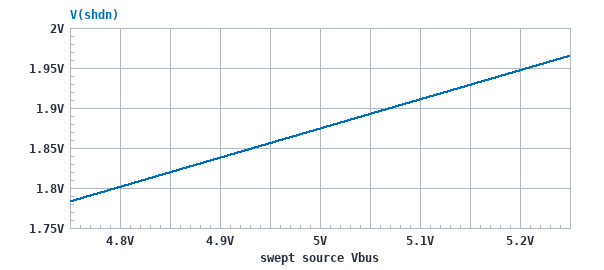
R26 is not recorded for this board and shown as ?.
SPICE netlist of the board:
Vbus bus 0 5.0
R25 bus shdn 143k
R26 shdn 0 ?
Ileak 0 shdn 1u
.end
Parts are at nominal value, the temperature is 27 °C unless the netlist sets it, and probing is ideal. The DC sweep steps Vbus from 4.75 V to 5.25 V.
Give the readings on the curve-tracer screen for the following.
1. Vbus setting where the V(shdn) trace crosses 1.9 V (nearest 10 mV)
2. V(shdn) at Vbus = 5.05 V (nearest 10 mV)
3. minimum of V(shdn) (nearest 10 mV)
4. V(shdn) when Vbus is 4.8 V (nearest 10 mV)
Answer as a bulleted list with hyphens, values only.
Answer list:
- 5.07 V
- 1.89 V
- 1.78 V
- 1.80 V
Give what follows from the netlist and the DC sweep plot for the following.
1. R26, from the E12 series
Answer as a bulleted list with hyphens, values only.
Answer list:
- 82 kΩ
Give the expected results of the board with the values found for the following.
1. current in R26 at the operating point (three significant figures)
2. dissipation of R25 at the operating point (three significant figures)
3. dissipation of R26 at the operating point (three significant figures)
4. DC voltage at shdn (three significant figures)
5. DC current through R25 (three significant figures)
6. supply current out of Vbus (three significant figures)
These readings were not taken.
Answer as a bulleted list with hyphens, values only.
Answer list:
- 22.9 µA
- 68.3 µW
- 42.8 µW
- 1.87 V
- 21.9 µA
- 21.9 µA
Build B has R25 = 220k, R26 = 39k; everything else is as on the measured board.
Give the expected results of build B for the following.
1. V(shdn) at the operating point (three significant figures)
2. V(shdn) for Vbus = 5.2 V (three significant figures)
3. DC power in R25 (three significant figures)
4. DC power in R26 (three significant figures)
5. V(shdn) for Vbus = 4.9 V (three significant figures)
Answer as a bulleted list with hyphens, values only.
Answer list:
- 786 mV
- 816 mV
- 80.7 µW
- 15.8 µW
- 771 mV
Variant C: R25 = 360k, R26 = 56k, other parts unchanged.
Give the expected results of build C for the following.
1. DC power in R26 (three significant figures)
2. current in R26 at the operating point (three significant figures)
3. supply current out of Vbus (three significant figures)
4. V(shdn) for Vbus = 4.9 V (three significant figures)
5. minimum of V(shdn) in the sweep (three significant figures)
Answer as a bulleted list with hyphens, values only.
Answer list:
- 9.30 µW
- 12.9 µA
- 11.9 µA
- 708 mV
- 688 mV
